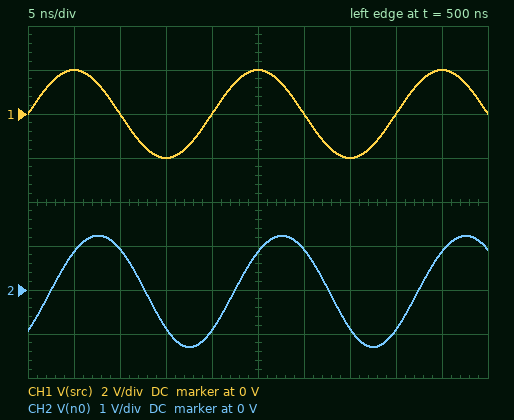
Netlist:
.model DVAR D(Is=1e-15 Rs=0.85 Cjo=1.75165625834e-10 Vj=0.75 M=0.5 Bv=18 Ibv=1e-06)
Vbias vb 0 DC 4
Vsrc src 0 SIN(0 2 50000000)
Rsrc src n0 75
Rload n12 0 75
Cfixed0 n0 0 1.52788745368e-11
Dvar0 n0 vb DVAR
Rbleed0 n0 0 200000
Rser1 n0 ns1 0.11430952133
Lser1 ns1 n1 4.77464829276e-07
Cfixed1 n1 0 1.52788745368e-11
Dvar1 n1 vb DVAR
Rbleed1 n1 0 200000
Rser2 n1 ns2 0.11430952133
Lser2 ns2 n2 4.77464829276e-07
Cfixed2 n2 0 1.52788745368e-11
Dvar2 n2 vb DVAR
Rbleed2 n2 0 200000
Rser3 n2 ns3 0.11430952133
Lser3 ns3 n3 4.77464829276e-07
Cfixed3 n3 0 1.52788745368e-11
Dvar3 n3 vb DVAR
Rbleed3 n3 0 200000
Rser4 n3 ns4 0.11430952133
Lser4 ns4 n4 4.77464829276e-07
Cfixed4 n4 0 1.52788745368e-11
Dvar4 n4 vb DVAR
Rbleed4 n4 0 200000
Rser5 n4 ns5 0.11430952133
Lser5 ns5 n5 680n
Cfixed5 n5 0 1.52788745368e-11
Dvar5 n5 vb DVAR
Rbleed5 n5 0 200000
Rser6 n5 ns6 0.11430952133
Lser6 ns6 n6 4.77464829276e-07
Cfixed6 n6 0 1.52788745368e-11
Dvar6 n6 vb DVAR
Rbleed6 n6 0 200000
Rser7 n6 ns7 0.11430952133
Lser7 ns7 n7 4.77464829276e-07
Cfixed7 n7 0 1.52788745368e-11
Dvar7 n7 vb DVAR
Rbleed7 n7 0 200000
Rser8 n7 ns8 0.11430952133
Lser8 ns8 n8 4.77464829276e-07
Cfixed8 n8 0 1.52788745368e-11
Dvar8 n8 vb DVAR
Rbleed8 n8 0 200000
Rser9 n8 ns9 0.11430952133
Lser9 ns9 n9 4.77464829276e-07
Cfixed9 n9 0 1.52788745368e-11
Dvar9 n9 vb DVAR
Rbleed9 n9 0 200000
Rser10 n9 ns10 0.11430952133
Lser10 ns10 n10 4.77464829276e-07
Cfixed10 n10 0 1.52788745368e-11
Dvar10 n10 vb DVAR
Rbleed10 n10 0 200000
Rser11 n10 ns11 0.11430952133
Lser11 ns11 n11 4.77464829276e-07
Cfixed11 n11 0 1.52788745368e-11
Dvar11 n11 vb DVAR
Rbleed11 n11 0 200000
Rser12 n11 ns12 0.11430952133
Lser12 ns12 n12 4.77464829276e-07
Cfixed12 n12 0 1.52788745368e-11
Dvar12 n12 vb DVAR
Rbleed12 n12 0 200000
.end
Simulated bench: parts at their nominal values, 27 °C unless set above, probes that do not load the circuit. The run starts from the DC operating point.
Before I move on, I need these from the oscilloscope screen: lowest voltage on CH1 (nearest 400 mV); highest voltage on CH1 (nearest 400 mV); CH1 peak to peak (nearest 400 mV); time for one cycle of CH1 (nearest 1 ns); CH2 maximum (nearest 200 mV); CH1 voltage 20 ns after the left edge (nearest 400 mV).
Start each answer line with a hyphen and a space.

- -2.0 V
- 2.0 V
- 4.0 V
- 20 ns
- 1.2 V
- 0 V
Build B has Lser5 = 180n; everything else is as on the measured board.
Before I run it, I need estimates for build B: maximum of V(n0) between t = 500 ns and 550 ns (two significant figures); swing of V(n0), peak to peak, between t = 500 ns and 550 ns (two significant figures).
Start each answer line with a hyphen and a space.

- 1.3 V
- 2.6 V
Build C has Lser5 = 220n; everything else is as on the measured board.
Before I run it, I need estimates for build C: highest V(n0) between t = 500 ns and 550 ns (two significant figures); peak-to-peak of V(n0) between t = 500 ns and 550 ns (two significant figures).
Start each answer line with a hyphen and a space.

- 1.3 V
- 2.6 V
